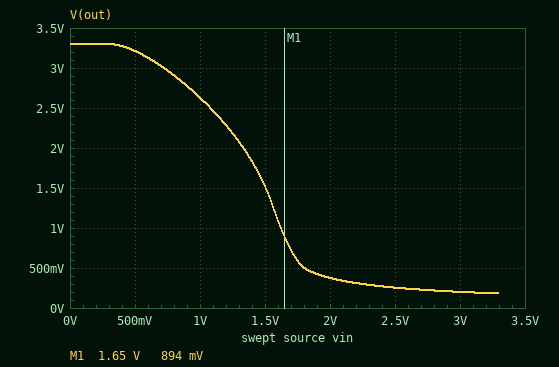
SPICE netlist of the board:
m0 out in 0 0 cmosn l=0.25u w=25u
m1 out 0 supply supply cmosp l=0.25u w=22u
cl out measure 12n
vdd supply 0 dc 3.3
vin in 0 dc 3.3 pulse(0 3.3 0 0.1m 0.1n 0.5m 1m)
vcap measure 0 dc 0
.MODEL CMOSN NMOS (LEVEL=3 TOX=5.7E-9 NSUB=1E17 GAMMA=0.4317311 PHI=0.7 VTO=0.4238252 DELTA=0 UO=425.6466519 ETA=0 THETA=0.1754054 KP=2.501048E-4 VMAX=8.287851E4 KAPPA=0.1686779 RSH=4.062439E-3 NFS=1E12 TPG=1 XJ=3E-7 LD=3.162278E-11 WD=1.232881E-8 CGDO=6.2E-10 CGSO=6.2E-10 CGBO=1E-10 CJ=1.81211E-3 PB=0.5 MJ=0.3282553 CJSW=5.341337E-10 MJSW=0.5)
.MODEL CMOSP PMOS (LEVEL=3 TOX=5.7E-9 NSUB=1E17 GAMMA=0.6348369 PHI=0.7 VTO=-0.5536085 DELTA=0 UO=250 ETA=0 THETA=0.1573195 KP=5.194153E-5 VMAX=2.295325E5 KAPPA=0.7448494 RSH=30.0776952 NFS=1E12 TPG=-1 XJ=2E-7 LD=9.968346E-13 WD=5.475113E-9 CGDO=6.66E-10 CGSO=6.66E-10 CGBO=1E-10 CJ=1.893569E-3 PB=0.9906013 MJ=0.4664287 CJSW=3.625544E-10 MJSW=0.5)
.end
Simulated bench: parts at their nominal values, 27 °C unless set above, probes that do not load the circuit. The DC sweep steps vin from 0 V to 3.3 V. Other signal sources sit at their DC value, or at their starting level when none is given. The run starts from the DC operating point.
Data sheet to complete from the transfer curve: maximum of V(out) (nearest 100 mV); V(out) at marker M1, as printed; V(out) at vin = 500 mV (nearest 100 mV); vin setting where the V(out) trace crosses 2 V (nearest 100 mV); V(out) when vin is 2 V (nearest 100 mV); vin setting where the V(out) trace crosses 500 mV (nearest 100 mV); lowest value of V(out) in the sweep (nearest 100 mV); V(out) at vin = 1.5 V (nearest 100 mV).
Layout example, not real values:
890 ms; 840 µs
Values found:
3.3 V; 894 mV; 3.2 V; 1.3 V; 400 mV; 1.8 V; 200 mV; 1.5 V
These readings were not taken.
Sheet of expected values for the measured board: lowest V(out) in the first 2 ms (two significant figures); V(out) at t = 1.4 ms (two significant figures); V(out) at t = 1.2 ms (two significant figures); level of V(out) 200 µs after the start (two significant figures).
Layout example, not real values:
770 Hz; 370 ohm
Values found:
180 mV; 180 mV; 180 mV; 180 mV
